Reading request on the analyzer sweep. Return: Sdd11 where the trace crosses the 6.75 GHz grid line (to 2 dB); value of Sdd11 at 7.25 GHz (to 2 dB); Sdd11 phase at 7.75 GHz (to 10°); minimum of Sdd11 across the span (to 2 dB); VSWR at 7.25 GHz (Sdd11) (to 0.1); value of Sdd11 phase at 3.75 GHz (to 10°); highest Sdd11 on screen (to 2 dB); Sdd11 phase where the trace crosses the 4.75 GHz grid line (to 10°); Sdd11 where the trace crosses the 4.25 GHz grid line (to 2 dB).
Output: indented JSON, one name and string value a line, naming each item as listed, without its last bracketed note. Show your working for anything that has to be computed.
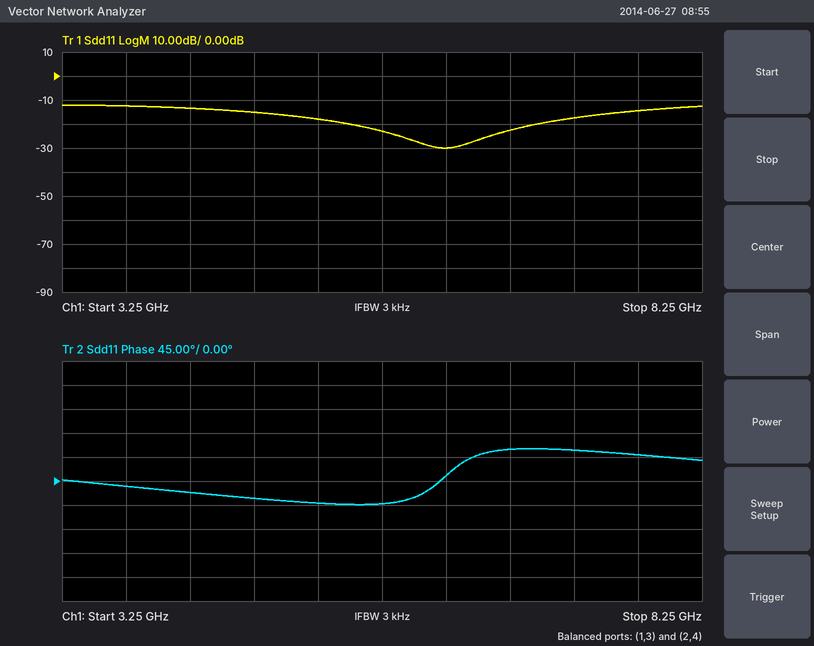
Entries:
{
  "Sdd11 where the trace crosses the 6.75 GHz grid line": "-22 dB",
  "value of Sdd11 at 7.25 GHz": "-18 dB",
  "Sdd11 phase at 7.75 GHz": "50°",
  "minimum of Sdd11 across the span": "-30 dB",
  "VSWR at 7.25 GHz (Sdd11)": "|Γ| = 10^(-18/20) = 0.1259; VSWR = (1 + 0.1259)/(1 − 0.1259) ≈ 1.3",
  "value of Sdd11 phase at 3.75 GHz": "-10°",
  "highest Sdd11 on screen": "-12 dB",
  "Sdd11 phase where the trace crosses the 4.75 GHz grid line": "-30°",
  "Sdd11 where the trace crosses the 4.25 GHz grid line": "-14 dB"
}
